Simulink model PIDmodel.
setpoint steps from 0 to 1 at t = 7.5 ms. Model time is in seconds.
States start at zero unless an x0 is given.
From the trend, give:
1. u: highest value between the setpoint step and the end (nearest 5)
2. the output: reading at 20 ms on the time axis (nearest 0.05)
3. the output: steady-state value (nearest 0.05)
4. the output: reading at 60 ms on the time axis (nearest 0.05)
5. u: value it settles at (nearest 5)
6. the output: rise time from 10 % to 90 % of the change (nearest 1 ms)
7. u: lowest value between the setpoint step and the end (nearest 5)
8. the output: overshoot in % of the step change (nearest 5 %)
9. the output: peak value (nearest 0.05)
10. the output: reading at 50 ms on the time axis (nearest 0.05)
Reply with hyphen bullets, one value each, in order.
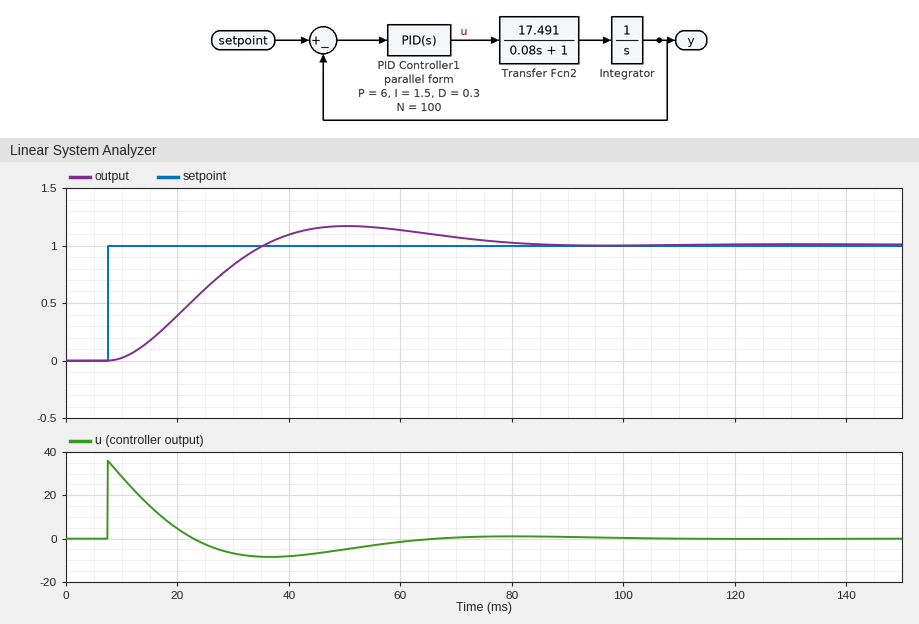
- 35
- 0.40
- 1.00
- 1.15
- 0
- 19 ms
- -10
- 15 %
- 1.15
- 1.15
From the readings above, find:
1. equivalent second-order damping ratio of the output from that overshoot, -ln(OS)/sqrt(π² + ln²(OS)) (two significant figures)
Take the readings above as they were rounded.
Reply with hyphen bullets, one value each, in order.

- 0.52
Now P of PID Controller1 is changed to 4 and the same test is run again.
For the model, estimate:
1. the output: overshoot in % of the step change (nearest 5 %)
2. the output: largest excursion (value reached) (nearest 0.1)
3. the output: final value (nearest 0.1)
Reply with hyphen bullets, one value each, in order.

- 10 %
- 1.1
- 1.0
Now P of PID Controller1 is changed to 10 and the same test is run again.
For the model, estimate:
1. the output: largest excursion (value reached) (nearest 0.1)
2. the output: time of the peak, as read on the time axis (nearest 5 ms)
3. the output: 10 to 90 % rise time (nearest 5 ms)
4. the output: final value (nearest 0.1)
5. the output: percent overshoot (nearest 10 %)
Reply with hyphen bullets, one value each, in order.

- 1.3
- 45 ms
- 15 ms
- 1.0
- 30 %
